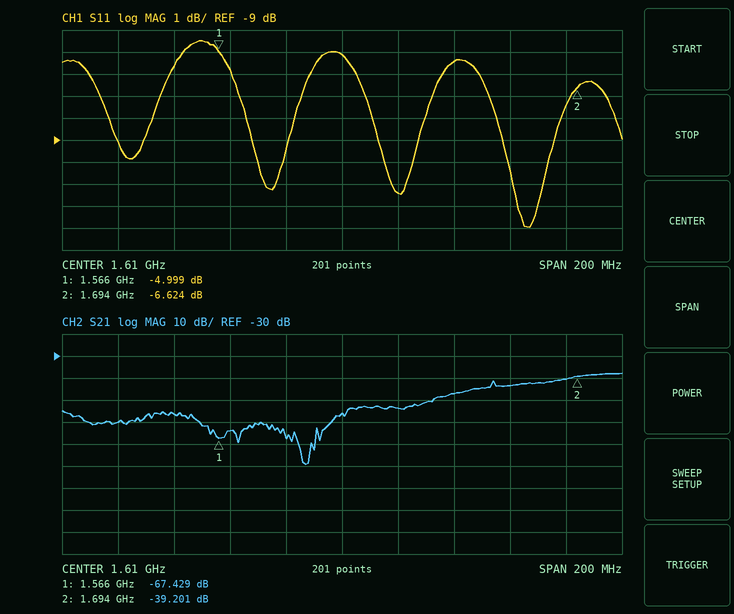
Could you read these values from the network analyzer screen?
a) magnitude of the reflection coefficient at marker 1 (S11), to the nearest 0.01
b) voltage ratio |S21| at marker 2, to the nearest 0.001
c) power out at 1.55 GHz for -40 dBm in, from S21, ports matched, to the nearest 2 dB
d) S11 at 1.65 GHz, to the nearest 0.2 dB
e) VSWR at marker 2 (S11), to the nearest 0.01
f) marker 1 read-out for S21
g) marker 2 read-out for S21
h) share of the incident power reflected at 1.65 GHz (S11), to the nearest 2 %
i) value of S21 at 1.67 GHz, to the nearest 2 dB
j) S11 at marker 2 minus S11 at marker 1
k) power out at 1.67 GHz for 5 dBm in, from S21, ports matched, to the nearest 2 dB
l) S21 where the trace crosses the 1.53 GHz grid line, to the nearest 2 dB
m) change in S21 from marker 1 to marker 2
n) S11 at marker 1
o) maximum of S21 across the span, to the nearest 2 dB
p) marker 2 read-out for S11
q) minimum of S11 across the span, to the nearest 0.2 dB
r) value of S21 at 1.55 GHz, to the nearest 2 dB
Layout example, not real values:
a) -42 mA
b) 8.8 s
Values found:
a) 0.56
b) 0.011
c) -96 dBm
d) -5.4 dB
e) 2.75
f) -67.429 dB
g) -39.201 dB
h) 28 %
i) -44 dB
j) -1.625 dB
k) -38 dBm
l) -60 dB
m) 28.228 dB
n) -4.999 dB
o) -38 dB
p) -6.624 dB
q) -13.0 dB
r) -56 dB
